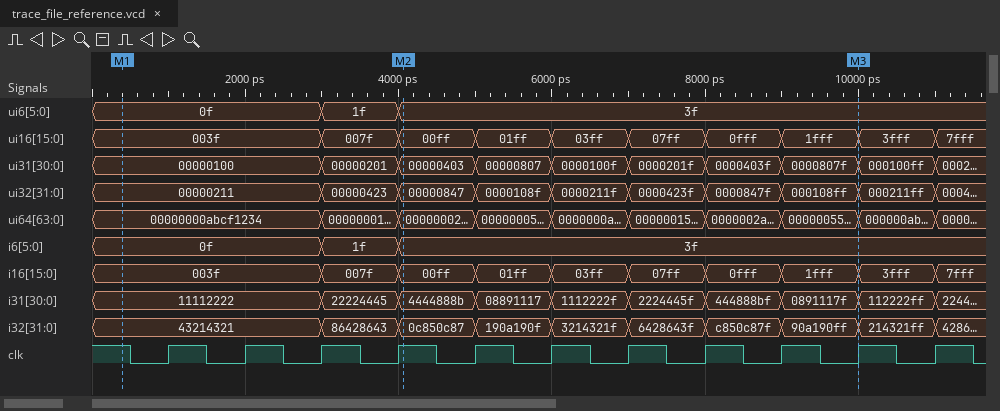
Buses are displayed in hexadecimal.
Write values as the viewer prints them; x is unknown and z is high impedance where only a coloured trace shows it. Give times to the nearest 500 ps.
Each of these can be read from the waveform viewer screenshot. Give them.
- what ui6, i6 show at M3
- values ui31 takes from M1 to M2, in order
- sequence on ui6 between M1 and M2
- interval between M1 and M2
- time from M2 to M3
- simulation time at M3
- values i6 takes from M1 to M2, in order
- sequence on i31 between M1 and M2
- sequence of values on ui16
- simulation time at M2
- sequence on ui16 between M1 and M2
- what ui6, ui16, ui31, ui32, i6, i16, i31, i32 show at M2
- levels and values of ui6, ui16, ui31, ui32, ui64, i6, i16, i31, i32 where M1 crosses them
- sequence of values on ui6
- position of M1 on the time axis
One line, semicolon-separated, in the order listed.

ui6=3f, i6=3f; 00000100, 00000201, 00000403; 0f, 1f, 3f; 3500 ps; 6000 ps; 10000 ps; 0f, 1f, 3f; 11112222, 22224445, 4444888b; 003f, 007f, 00ff, 01ff, 03ff, 07ff, 0fff, 1fff, 3fff, 7fff; 4000 ps; 003f, 007f, 00ff; ui6=3f, ui16=00ff, ui31=00000403, ui32=00000847, i6=3f, i16=00ff, i31=4444888b, i32=0c850c87; ui6=0f, ui16=003f, ui31=00000100, ui32=00000211, ui64=00000000abcf1234, i6=0f, i16=003f, i31=11112222, i32=43214321; 0f, 1f, 3f; 500 ps
